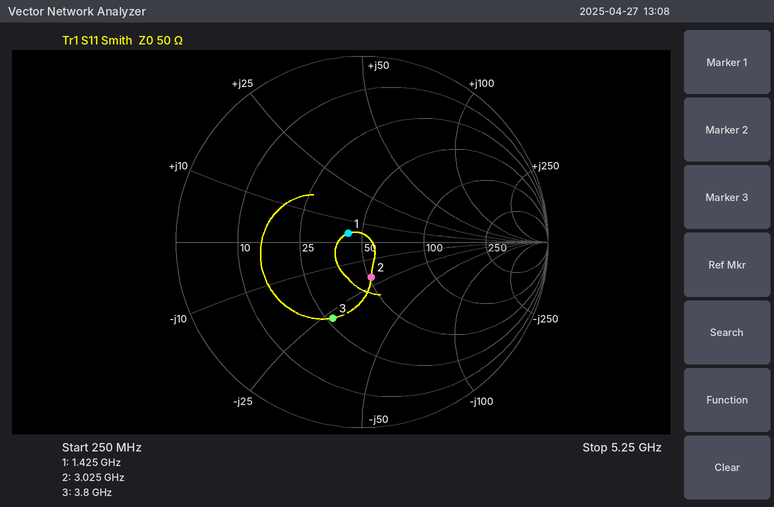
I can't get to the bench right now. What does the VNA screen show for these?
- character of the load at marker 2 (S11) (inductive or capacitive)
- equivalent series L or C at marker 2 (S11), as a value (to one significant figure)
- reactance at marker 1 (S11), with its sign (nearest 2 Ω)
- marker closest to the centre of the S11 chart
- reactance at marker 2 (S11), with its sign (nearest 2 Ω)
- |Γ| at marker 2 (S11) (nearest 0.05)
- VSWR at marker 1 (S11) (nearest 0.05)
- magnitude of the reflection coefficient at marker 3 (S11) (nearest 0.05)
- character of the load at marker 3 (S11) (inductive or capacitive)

capacitive
3 pF
+4 Ω
marker 1
-20 Ω
0.20
1.20
0.45
capacitive
